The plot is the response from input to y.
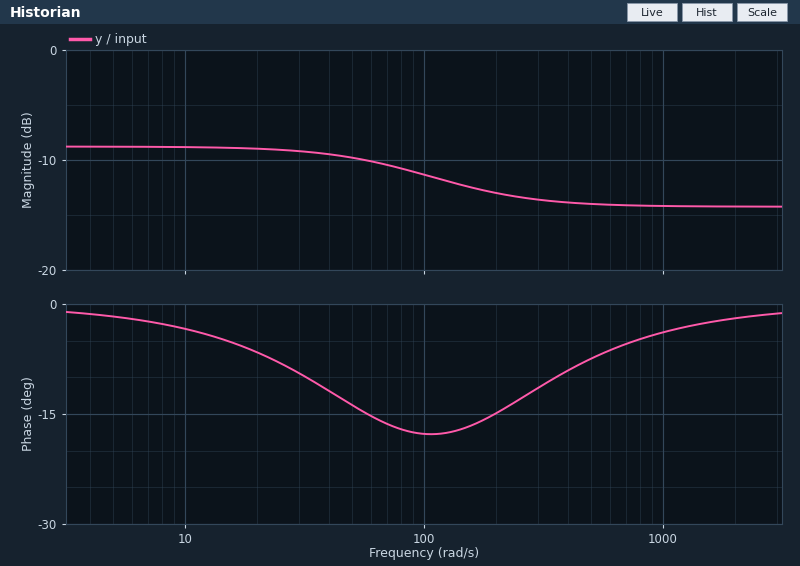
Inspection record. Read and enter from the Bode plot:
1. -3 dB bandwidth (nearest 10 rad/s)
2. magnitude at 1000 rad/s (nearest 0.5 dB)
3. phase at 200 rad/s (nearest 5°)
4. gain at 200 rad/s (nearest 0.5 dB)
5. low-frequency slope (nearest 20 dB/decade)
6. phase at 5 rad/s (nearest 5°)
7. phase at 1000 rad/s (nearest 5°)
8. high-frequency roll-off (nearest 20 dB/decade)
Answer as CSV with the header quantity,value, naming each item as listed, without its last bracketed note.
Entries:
quantity,value
-3 dB bandwidth,120 rad/s
magnitude at 1000 rad/s,-14.0 dB
phase at 200 rad/s,-15°
gain at 200 rad/s,-13.0 dB
low-frequency slope,0 dB/decade
phase at 5 rad/s,0°
phase at 1000 rad/s,-5°
high-frequency roll-off,0 dB/decade
